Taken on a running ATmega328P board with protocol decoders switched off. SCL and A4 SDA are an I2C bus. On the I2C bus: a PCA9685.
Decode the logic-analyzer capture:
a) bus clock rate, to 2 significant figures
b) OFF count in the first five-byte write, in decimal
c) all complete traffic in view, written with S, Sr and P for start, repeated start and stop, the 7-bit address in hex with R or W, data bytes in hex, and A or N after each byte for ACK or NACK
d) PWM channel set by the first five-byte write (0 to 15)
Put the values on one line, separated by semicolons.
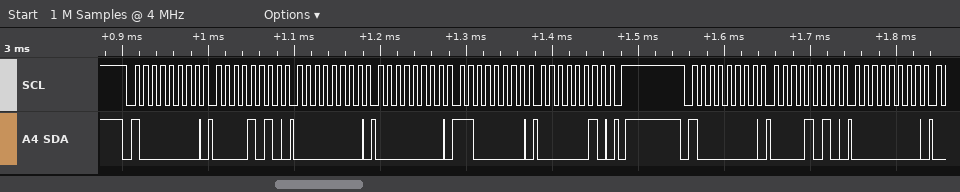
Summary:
100 kHz; 704; S 40W A 0A A 00 A 00 A C0 A 02 A P S 40W A 0A A 00 A; 1
